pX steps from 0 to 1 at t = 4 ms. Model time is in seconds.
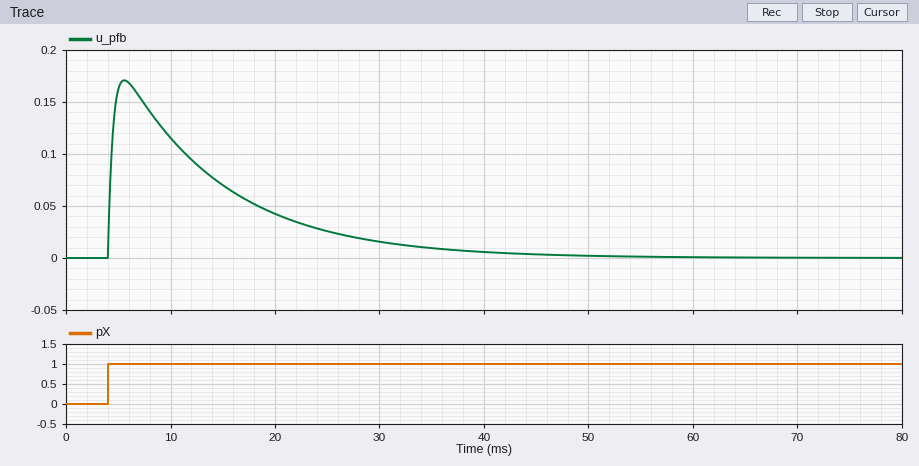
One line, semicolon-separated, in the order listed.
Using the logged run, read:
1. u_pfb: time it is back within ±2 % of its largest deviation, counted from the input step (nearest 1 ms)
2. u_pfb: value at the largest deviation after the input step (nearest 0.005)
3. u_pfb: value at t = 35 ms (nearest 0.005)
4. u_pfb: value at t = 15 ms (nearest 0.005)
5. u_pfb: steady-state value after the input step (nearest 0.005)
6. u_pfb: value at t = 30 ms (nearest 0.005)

41 ms; 0.170; 0.010; 0.070; 0.000; 0.015
